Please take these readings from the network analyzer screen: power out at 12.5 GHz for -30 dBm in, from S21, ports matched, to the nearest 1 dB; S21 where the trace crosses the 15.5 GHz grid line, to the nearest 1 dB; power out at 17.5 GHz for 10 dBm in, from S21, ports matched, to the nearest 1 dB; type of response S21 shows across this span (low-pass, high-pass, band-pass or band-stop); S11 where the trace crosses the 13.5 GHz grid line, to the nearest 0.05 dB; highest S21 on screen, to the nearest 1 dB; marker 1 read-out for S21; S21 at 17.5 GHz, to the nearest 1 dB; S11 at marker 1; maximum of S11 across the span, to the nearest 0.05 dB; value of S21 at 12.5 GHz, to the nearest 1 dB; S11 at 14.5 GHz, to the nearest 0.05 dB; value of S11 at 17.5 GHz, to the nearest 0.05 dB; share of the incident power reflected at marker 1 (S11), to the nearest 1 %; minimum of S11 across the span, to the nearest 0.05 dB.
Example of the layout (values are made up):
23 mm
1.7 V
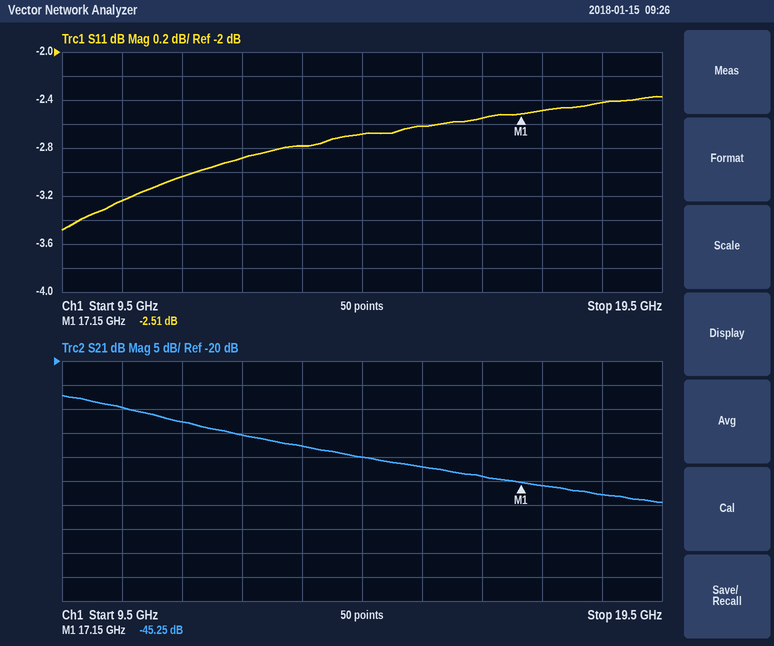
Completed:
-65 dBm
-42 dB
-36 dBm
low-pass
-2.80 dB
-27 dB
-45.25 dB
-46 dB
-2.51 dB
-2.35 dB
-35 dB
-2.70 dB
-2.50 dB
56 %
-3.50 dB
